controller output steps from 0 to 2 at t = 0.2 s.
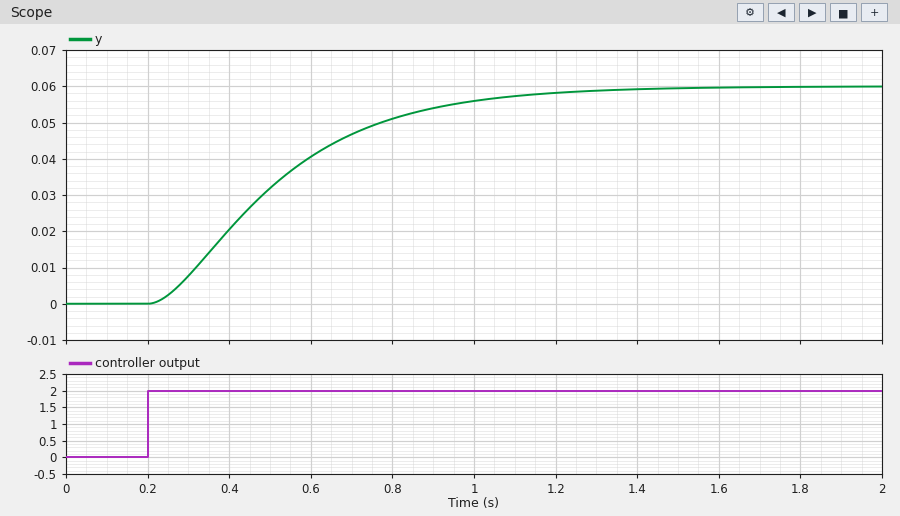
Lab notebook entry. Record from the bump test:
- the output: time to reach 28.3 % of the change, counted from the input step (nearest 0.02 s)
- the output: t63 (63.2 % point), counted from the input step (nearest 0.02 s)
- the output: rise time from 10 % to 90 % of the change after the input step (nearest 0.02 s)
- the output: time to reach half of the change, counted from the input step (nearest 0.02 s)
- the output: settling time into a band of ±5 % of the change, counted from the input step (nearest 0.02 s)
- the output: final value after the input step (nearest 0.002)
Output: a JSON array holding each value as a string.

["0.18 s", "0.36 s", "0.62 s", "0.28 s", "0.88 s", "0.060"]
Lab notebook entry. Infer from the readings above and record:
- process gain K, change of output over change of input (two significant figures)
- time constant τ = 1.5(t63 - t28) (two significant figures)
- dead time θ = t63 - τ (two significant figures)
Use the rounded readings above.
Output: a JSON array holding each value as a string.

["0.030", "0.27 s", "0.090 s"]
